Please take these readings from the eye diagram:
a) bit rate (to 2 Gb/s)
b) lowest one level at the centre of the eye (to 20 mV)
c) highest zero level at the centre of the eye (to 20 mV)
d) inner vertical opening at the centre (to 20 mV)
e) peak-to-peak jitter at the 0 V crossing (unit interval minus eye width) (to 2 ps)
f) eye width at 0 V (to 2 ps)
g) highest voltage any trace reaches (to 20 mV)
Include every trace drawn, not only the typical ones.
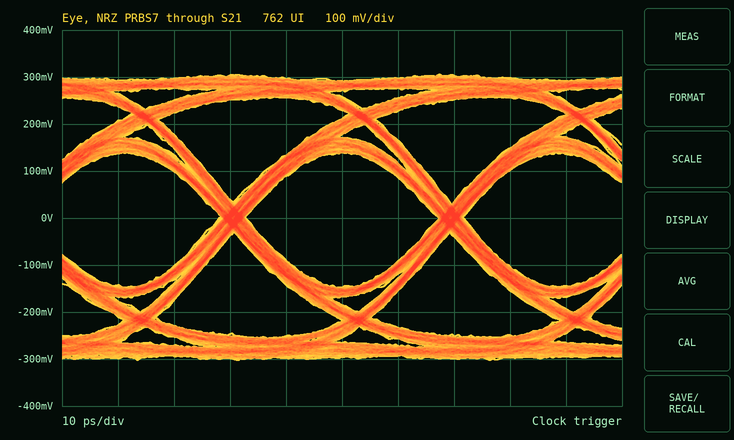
26 Gb/s
140 mV
-140 mV
280 mV
4 ps
34 ps
300 mV
